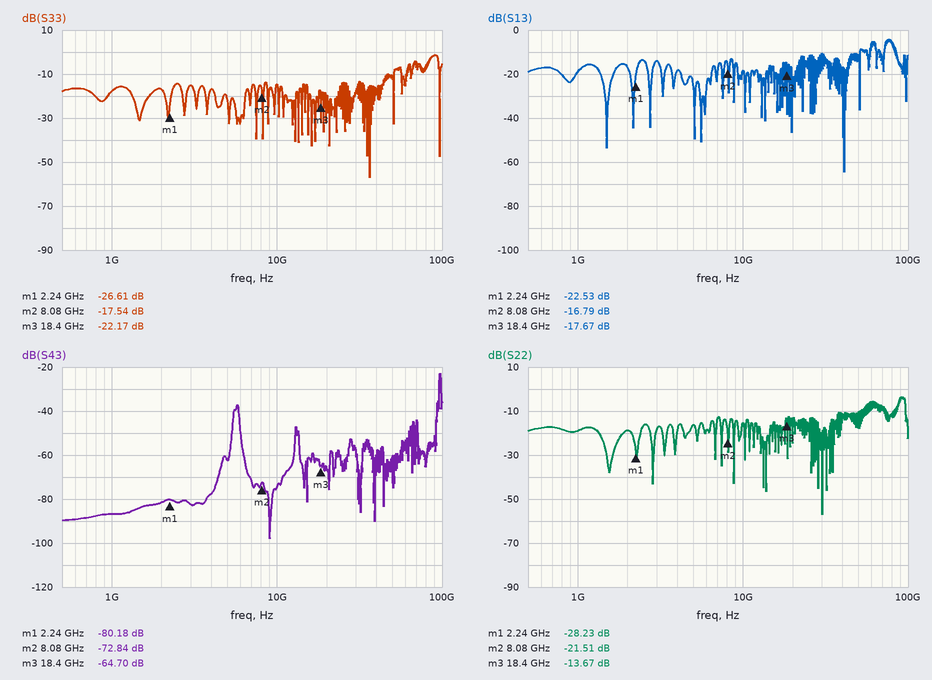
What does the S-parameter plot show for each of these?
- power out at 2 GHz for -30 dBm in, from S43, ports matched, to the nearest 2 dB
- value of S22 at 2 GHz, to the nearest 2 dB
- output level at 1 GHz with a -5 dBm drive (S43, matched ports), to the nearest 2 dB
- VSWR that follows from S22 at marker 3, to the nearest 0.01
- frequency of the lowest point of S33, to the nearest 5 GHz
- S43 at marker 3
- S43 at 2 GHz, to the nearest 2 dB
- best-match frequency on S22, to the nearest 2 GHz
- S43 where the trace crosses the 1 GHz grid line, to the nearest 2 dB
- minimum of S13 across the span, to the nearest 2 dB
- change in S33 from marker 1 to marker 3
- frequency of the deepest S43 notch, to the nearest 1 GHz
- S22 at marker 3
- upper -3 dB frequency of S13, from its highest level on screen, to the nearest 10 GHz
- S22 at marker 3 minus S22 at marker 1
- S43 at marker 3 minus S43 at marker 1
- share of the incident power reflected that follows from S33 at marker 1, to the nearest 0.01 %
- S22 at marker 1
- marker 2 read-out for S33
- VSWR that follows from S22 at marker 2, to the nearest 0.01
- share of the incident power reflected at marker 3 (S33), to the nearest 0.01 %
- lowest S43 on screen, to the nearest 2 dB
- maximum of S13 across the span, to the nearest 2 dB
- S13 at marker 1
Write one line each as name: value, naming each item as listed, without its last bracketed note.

power out at 2 GHz for -30 dBm in, from S43, ports matched, to the nearest 2 dB: -112 dBm
value of S22 at 2 GHz, to the nearest 2 dB: -18 dB
output level at 1 GHz with a -5 dBm drive (S43, matched ports), to the nearest 2 dB: -92 dBm
VSWR that follows from S22 at marker 3, to the nearest 0.01: 1.52
frequency of the lowest point of S33, to the nearest 5 GHz: 35 GHz
S43 at marker 3: -64.70 dB
S43 at 2 GHz, to the nearest 2 dB: -82 dB
best-match frequency on S22, to the nearest 2 GHz: 30 GHz
S43 where the trace crosses the 1 GHz grid line, to the nearest 2 dB: -86 dB
minimum of S13 across the span, to the nearest 2 dB: -64 dB
change in S33 from marker 1 to marker 3: 4.44 dB
frequency of the deepest S43 notch, to the nearest 1 GHz: 9 GHz
S22 at marker 3: -13.67 dB
upper -3 dB frequency of S13, from its highest level on screen, to the nearest 10 GHz: 80 GHz
S22 at marker 3 minus S22 at marker 1: 14.56 dB
S43 at marker 3 minus S43 at marker 1: 15.48 dB
share of the incident power reflected that follows from S33 at marker 1, to the nearest 0.01 %: 0.22 %
S22 at marker 1: -28.23 dB
marker 2 read-out for S33: -17.54 dB
VSWR that follows from S22 at marker 2, to the nearest 0.01: 1.18
share of the incident power reflected at marker 3 (S33), to the nearest 0.01 %: 0.61 %
lowest S43 on screen, to the nearest 2 dB: -98 dB
maximum of S13 across the span, to the nearest 2 dB: -4 dB
S13 at marker 1: -22.53 dB
